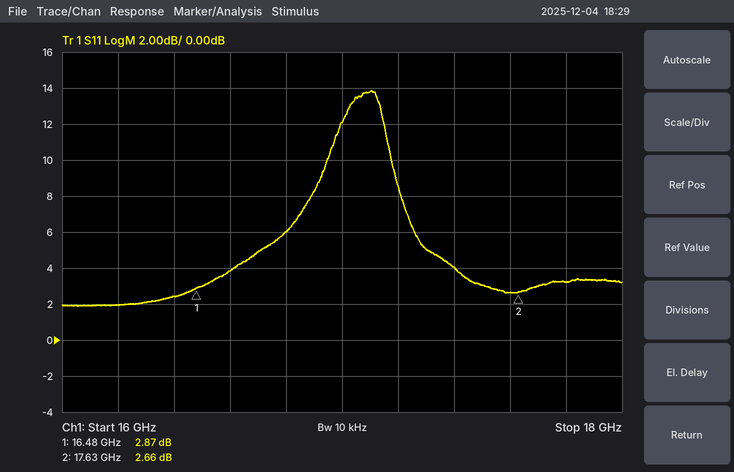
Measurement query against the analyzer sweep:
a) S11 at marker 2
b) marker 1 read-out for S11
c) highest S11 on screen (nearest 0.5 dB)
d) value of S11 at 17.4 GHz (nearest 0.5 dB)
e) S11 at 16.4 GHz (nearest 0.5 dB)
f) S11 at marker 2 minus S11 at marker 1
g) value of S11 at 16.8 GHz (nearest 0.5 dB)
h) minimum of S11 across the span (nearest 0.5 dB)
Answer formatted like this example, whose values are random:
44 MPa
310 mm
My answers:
2.66 dB
2.87 dB
14.0 dB
4.0 dB
2.5 dB
-0.21 dB
6.0 dB
2.0 dB
